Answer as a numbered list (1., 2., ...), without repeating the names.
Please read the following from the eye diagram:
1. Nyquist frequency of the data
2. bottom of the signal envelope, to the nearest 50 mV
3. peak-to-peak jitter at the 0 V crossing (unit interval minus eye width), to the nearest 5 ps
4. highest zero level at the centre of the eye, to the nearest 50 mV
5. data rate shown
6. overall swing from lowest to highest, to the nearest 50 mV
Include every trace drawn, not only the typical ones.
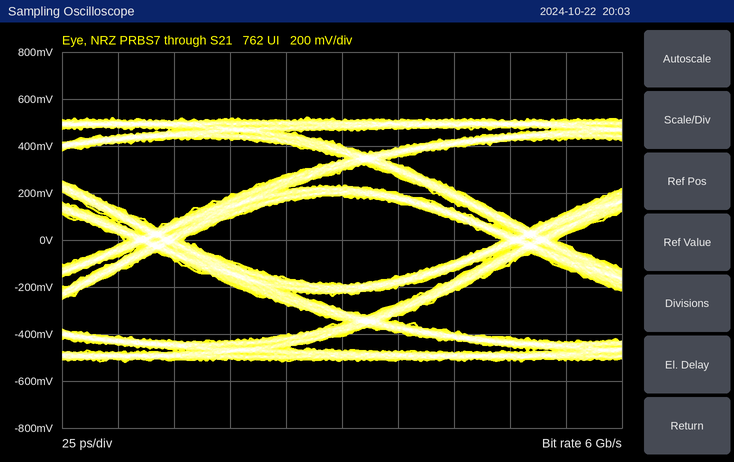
1. 3 GHz
2. -500 mV
3. 25 ps
4. -200 mV
5. 6 Gb/s
6. 1.05 V
